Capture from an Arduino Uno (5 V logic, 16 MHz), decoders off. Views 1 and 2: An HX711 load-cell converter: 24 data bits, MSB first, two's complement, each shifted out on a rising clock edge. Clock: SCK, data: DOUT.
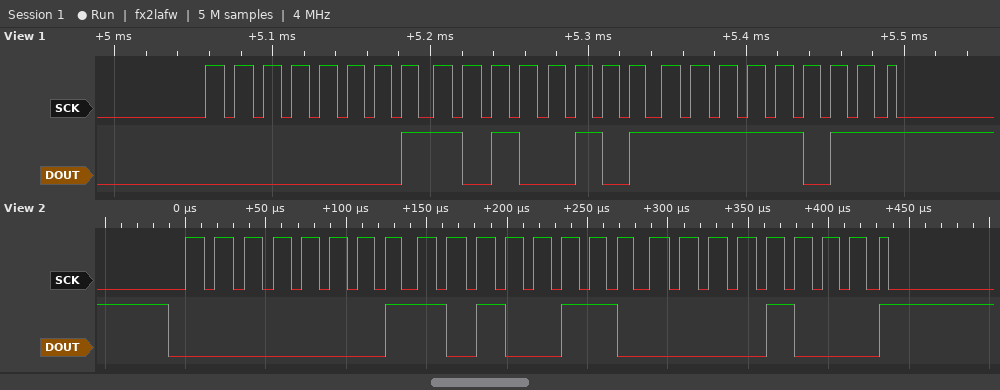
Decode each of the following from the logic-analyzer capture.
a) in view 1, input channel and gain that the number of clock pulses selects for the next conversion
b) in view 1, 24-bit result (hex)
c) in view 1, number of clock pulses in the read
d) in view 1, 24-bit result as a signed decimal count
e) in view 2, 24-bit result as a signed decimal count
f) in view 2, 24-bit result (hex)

channel A, gain 128
0x01A5FB
25
108027
108040
0x01A608
